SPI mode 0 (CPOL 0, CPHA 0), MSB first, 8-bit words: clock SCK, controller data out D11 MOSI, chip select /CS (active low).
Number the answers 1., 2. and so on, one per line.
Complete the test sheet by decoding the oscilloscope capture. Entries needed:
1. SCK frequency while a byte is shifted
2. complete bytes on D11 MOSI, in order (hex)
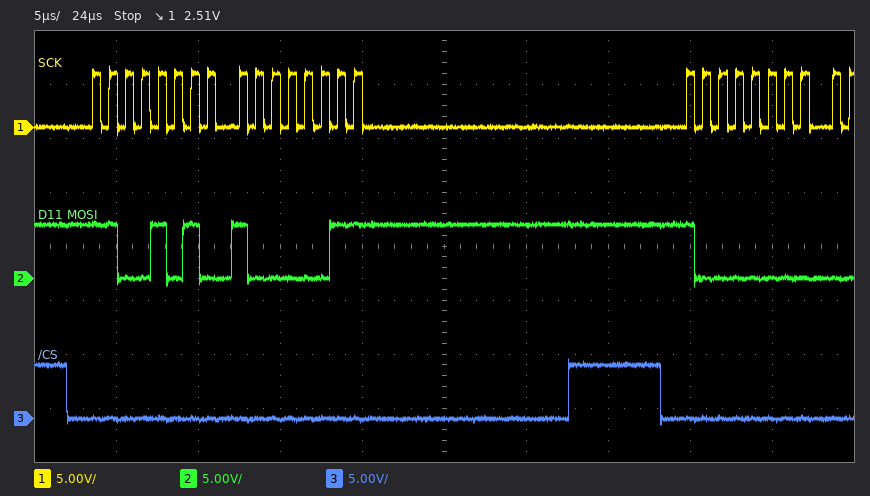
1. 1 MHz
2. CA 83 80
